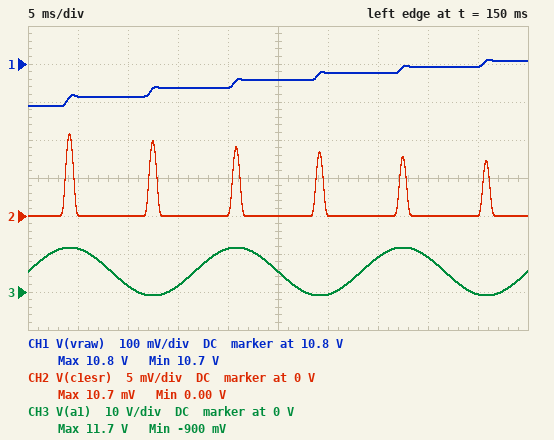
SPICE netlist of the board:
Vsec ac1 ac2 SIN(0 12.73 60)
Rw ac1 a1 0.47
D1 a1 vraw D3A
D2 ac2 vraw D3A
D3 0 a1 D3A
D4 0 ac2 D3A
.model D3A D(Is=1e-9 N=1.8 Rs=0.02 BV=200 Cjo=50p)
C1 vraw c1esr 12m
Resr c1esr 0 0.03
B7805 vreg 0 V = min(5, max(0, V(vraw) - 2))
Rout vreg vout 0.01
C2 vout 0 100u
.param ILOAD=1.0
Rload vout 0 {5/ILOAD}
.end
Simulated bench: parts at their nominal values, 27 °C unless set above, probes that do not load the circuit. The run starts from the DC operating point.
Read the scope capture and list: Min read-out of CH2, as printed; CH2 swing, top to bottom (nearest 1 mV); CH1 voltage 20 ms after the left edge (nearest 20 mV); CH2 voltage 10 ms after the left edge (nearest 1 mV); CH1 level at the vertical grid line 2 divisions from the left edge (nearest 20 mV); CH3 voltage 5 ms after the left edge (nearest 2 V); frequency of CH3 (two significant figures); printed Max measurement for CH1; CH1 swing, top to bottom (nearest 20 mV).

0.00 V
11 mV
10.74 V
0 V
10.72 V
12 V
60 Hz
10.8 V
120 mV
